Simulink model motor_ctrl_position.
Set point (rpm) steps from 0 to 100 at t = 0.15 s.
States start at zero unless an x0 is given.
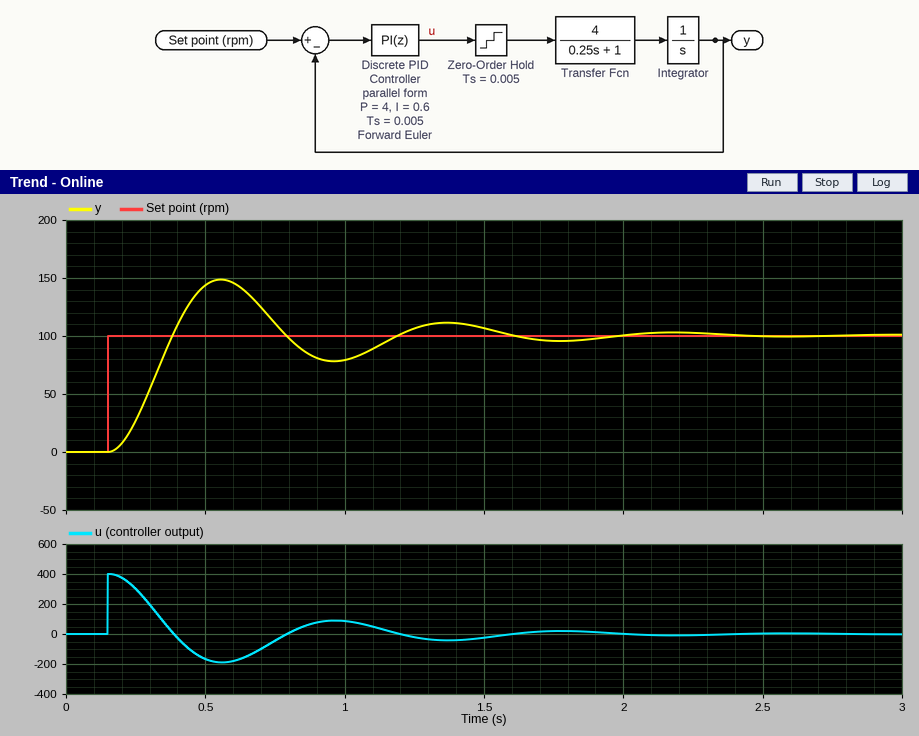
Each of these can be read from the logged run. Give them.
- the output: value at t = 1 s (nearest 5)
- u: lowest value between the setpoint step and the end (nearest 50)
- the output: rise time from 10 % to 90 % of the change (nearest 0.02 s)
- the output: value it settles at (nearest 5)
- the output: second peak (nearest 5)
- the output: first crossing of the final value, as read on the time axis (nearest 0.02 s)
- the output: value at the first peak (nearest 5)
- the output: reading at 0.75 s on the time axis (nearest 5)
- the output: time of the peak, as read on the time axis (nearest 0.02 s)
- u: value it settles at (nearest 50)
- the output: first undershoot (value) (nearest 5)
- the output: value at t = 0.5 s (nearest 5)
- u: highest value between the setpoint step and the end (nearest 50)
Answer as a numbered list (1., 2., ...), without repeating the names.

1. 80
2. -200
3. 0.16 s
4. 100
5. 110
6. 0.38 s
7. 150
8. 110
9. 0.56 s
10. 0
11. 80
12. 145
13. 400
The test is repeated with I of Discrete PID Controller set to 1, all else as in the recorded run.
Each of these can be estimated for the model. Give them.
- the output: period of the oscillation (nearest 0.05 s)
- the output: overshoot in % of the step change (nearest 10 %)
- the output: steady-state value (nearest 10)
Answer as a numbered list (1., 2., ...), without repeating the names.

1. 0.80 s
2. 50 %
3. 100
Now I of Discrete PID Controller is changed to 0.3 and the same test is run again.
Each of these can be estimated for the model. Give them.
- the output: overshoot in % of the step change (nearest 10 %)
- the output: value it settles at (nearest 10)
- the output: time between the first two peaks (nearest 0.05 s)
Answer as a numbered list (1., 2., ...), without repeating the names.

1. 50 %
2. 100
3. 0.80 s
